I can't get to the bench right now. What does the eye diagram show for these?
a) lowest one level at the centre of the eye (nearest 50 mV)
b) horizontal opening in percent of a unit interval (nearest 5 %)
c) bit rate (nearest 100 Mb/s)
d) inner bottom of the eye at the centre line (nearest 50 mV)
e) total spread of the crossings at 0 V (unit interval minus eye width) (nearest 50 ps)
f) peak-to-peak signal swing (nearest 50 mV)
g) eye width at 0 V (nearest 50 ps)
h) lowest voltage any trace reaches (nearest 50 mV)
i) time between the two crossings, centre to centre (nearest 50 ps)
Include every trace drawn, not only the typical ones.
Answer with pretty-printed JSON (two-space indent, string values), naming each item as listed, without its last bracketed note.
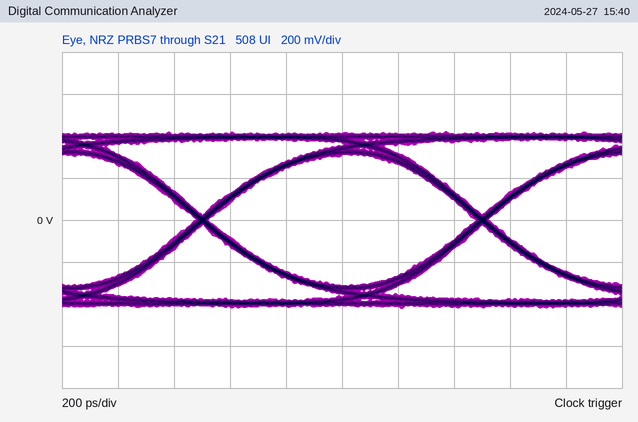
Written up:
{
  "lowest one level at the centre of the eye": "300 mV",
  "horizontal opening in percent of a unit interval": "95 %",
  "bit rate": "1.0 Gb/s",
  "inner bottom of the eye at the centre line": "-300 mV",
  "total spread of the crossings at 0 V (unit interval minus eye width)": "50 ps",
  "peak-to-peak signal swing": "850 mV",
  "eye width at 0 V": "950 ps",
  "lowest voltage any trace reaches": "-400 mV",
  "time between the two crossings, centre to centre": "1.00 ns"
}
